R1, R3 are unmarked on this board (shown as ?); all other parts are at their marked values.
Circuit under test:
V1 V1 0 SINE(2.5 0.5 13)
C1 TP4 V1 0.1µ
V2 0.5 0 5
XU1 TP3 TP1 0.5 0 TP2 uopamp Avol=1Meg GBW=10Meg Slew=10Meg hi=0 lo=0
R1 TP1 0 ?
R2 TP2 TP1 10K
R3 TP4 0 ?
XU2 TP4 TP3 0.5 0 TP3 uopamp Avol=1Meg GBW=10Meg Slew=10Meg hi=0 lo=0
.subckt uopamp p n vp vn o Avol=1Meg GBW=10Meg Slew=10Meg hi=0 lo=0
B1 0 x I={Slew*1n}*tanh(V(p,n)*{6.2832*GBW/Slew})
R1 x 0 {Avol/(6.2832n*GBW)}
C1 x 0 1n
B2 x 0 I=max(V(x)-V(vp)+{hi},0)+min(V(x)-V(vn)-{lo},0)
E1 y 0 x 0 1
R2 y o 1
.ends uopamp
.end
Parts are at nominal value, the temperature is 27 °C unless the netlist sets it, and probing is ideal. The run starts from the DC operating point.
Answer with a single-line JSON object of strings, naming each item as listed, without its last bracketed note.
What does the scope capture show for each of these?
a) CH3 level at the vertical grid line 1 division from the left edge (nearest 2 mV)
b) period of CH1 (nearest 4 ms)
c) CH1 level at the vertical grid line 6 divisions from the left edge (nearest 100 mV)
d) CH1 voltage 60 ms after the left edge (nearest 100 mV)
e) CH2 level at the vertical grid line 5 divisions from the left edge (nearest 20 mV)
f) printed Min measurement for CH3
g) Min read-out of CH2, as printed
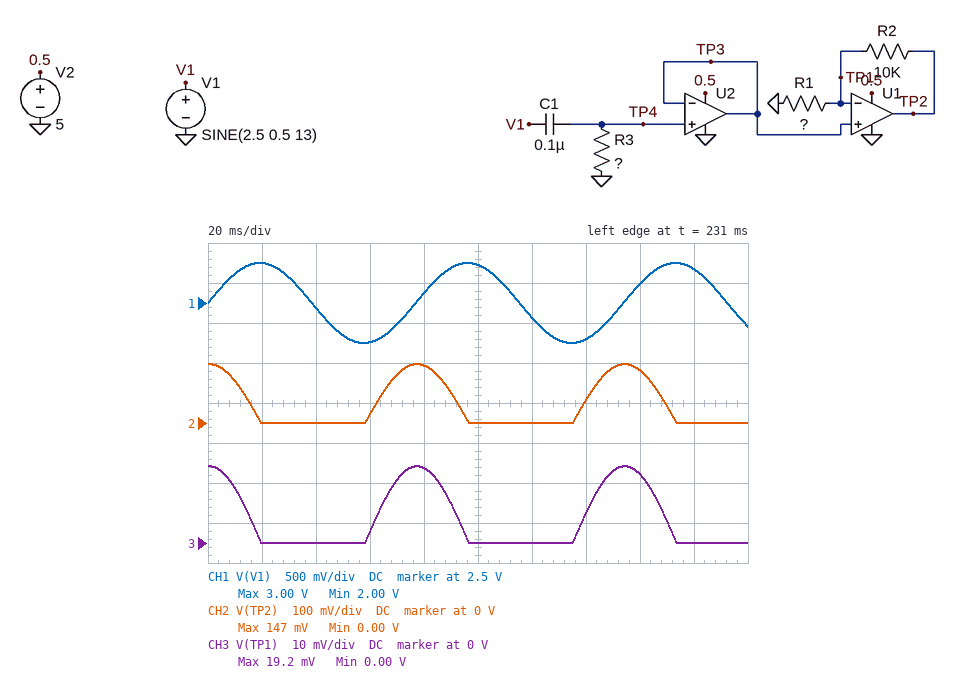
{"CH3 level at the vertical grid line 1 division from the left edge": "0 V", "period of CH1": "76 ms", "CH1 level at the vertical grid line 6 divisions from the left edge": "2.3 V", "CH1 voltage 60 ms after the left edge": "2.0 V", "CH2 level at the vertical grid line 5 divisions from the left edge": "0 V", "printed Min measurement for CH3": "0.00 V", "Min read-out of CH2, as printed": "0.00 V"}
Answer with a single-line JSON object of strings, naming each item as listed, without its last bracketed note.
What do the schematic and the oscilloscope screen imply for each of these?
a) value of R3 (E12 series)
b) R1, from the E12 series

{"value of R3": "4.7 kΩ", "R1, from the E12 series": "1.5 kΩ"}
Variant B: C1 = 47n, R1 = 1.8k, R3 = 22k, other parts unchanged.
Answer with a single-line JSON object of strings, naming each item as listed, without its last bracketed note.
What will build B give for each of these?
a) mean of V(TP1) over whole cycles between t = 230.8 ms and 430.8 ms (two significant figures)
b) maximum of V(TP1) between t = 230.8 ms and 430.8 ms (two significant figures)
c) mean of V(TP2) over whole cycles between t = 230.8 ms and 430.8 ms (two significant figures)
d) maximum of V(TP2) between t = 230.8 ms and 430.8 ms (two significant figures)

{"mean of V(TP1) over whole cycles between t = 230.8 ms and 430.8 ms": "13 mV", "maximum of V(TP1) between t = 230.8 ms and 430.8 ms": "42 mV", "mean of V(TP2) over whole cycles between t = 230.8 ms and 430.8 ms": "88 mV", "maximum of V(TP2) between t = 230.8 ms and 430.8 ms": "280 mV"}
